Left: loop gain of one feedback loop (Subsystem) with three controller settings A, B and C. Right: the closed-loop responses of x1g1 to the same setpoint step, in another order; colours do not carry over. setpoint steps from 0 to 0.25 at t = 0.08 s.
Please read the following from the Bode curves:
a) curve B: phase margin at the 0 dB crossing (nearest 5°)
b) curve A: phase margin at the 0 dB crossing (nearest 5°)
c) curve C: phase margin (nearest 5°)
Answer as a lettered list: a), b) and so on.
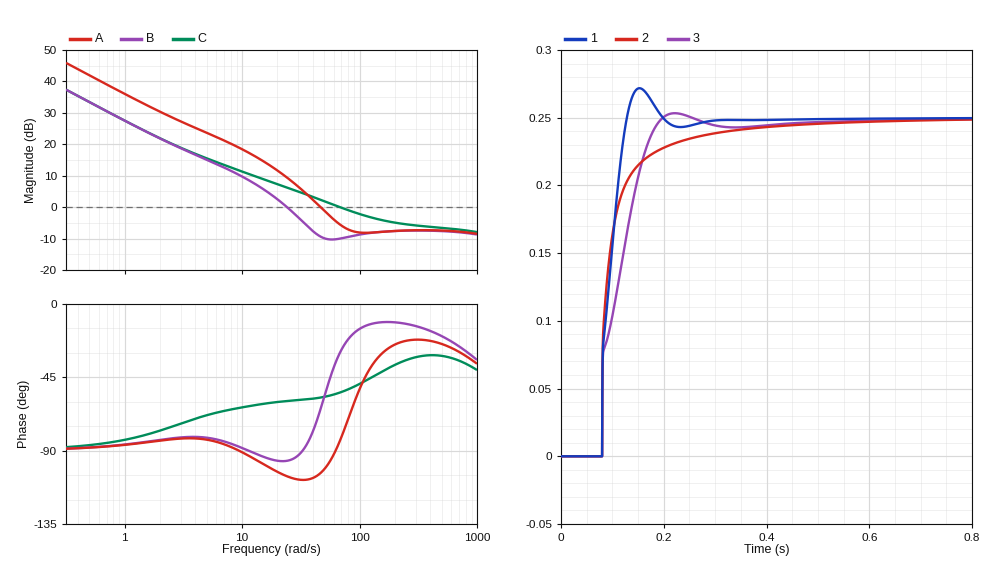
a) 85°
b) 75°
c) 125°
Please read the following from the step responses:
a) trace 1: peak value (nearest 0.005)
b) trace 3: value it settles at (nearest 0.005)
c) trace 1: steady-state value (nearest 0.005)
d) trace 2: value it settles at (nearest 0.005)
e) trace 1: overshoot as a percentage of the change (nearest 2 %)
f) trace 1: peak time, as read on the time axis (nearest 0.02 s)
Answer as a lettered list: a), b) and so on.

a) 0.270
b) 0.250
c) 0.250
d) 0.250
e) 8 %
f) 0.16 s
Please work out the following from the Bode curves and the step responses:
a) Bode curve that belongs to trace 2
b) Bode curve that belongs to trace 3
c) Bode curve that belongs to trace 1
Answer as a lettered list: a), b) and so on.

a) C
b) B
c) A
